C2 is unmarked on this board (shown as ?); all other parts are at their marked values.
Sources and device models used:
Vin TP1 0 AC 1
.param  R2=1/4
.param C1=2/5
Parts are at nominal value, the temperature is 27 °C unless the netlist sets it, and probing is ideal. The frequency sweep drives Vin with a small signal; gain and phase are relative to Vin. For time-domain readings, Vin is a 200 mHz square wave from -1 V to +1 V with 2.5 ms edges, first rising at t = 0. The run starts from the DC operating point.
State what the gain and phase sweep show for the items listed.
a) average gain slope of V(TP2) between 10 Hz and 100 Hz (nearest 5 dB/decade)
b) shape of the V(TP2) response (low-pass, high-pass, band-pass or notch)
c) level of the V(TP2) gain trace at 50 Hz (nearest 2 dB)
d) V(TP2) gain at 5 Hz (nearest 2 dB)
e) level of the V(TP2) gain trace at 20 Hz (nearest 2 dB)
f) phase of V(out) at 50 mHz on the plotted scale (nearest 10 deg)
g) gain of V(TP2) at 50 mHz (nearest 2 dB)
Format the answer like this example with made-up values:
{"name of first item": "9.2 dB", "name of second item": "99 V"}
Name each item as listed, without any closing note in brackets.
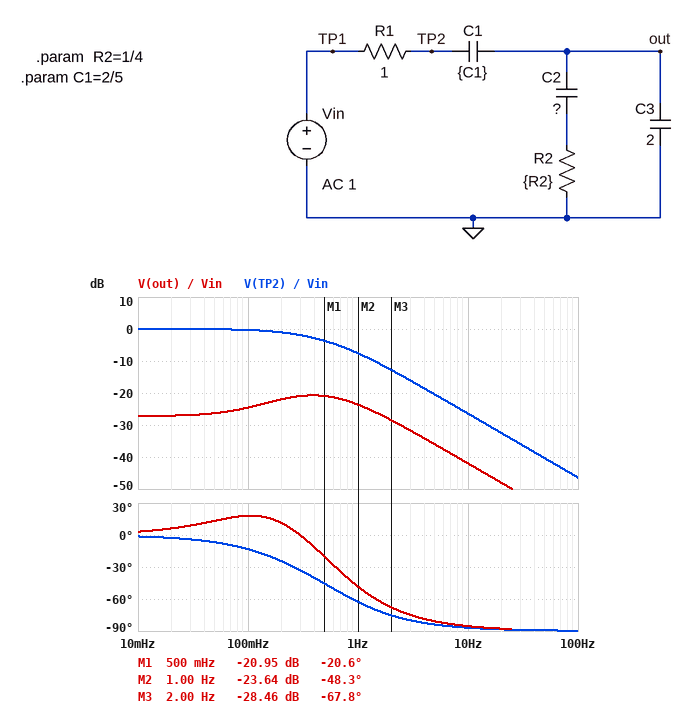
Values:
{"average gain slope of V(TP2) between 10 Hz and 100 Hz": "-20 dB/decade", "shape of the V(TP2) response": "low-pass", "level of the V(TP2) gain trace at 50 Hz": "-40 dB", "V(TP2) gain at 5 Hz": "-20 dB", "level of the V(TP2) gain trace at 20 Hz": "-32 dB", "phase of V(out) at 50 mHz on the plotted scale": "10 deg", "gain of V(TP2) at 50 mHz": "0 dB"}
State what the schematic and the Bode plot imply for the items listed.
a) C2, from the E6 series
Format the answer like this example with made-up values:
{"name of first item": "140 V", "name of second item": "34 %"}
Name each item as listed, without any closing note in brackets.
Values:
{"C2, from the E6 series": "6.8 F"}
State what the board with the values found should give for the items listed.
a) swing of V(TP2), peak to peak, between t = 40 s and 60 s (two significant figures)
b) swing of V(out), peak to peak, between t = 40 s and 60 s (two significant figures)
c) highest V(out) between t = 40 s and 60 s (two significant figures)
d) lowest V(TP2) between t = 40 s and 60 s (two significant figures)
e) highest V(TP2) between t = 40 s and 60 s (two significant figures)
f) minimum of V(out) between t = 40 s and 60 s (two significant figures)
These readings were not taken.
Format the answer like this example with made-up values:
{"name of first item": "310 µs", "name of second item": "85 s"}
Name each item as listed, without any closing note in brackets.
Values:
{"swing of V(TP2), peak to peak, between t = 40 s and 60 s": "2.0 V", "swing of V(out), peak to peak, between t = 40 s and 60 s": "230 mV", "highest V(out) between t = 40 s and 60 s": "160 mV", "lowest V(TP2) between t = 40 s and 60 s": "-990 mV", "highest V(TP2) between t = 40 s and 60 s": "990 mV", "minimum of V(out) between t = 40 s and 60 s": "-72 mV"}
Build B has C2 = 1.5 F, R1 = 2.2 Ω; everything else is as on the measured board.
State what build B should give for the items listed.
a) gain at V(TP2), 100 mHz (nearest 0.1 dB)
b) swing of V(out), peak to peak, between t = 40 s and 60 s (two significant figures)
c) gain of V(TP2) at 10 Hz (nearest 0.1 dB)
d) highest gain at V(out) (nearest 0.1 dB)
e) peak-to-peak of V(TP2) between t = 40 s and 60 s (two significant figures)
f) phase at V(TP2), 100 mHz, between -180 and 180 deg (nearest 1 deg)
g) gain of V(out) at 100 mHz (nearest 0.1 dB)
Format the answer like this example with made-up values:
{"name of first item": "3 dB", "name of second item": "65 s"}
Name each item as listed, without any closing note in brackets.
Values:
{"gain at V(TP2), 100 mHz": "-1.0 dB", "swing of V(out), peak to peak, between t = 40 s and 60 s": "190 mV", "gain of V(TP2) at 10 Hz": "-33.3 dB", "highest gain at V(out)": "-19.8 dB", "peak-to-peak of V(TP2) between t = 40 s and 60 s": "1.8 V", "phase at V(TP2), 100 mHz, between -180 and 180 deg": "-26 deg", "gain of V(out) at 100 mHz": "-20.6 dB"}
